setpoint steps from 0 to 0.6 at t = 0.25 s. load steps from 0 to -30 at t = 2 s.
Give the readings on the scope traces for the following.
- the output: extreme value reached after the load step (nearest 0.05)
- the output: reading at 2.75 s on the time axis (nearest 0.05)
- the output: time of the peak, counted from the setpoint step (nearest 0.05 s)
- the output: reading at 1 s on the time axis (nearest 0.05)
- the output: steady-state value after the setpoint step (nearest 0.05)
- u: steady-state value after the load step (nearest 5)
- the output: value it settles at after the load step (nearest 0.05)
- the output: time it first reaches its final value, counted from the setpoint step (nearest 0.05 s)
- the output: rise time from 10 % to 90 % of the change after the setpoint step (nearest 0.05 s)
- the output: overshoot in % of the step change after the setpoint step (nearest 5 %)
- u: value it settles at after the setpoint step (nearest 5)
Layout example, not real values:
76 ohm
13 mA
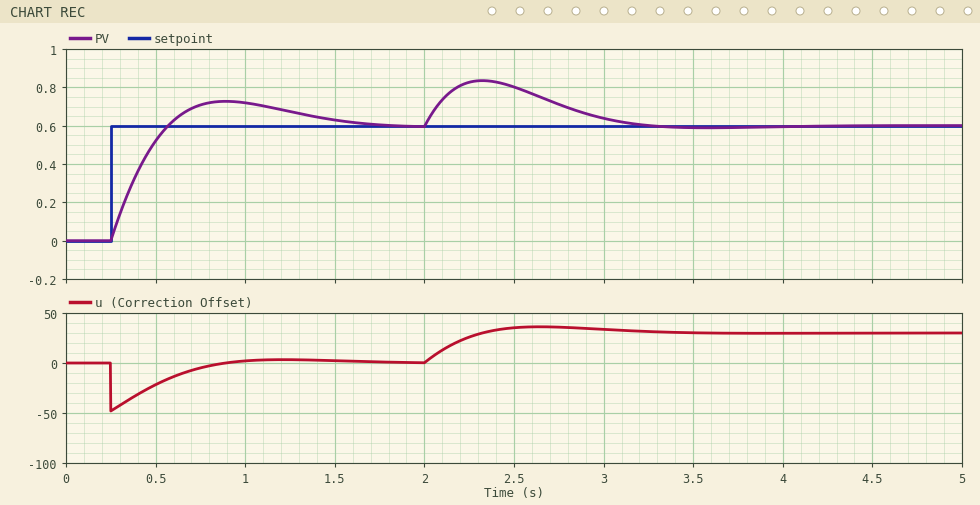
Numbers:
0.85
0.70
0.65 s
0.70
0.60
30
0.60
0.30 s
0.25 s
20 %
0
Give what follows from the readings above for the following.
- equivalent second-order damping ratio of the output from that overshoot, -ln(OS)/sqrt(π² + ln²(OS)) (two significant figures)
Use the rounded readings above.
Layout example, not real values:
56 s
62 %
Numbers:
0.46
